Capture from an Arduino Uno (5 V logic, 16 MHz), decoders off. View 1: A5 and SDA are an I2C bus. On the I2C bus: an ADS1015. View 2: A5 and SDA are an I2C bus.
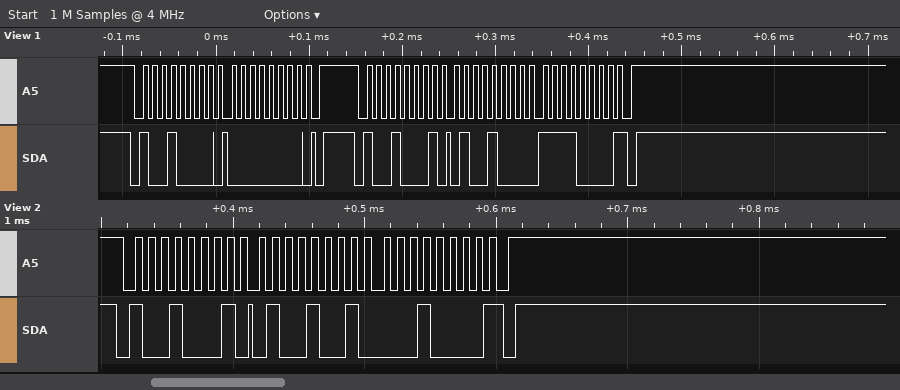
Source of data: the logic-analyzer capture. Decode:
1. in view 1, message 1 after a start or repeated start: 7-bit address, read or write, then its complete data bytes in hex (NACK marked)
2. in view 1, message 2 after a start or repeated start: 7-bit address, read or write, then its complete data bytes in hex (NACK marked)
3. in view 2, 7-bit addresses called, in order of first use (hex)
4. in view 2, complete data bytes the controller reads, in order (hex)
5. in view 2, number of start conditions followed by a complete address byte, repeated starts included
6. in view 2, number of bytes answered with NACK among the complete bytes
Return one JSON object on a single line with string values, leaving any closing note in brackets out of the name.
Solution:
{"in view 1, message 1 after a start or repeated start: 7-bit address, read or write, then its complete data bytes in hex": "0x48 write: 00", "in view 1, message 2 after a start or repeated start: 7-bit address, read or write, then its complete data bytes in hex": "0x48 read: 48 F0 NACK", "in view 2, 7-bit addresses called, in order of first use": "0x48", "in view 2, complete data bytes the controller reads, in order": "49 10", "in view 2, number of start conditions followed by a complete address byte, repeated starts included": "1", "in view 2, number of bytes answered with NACK among the complete bytes": "1"}
